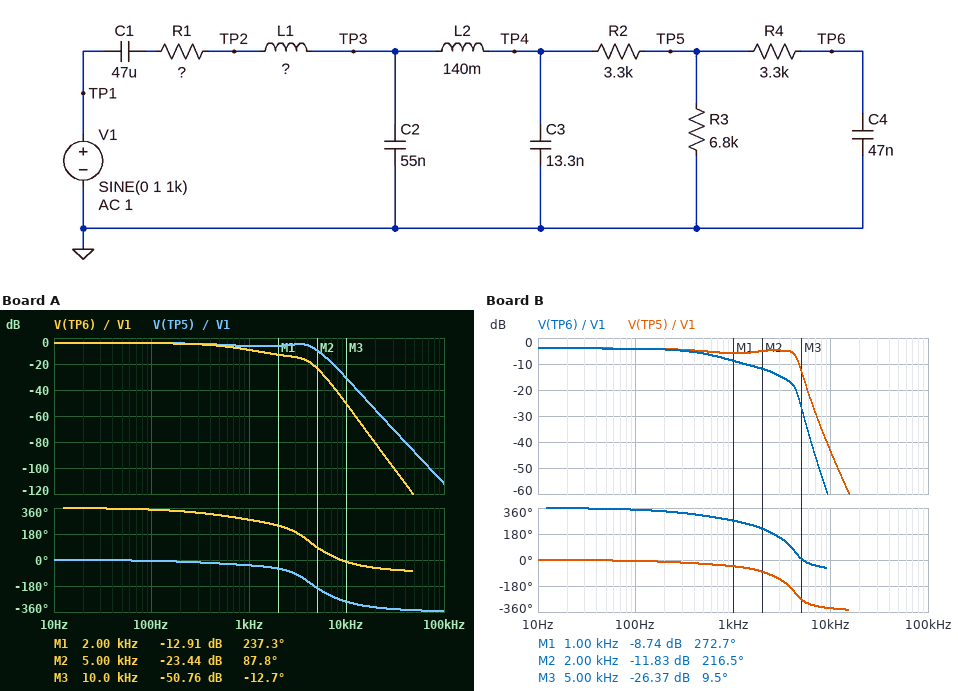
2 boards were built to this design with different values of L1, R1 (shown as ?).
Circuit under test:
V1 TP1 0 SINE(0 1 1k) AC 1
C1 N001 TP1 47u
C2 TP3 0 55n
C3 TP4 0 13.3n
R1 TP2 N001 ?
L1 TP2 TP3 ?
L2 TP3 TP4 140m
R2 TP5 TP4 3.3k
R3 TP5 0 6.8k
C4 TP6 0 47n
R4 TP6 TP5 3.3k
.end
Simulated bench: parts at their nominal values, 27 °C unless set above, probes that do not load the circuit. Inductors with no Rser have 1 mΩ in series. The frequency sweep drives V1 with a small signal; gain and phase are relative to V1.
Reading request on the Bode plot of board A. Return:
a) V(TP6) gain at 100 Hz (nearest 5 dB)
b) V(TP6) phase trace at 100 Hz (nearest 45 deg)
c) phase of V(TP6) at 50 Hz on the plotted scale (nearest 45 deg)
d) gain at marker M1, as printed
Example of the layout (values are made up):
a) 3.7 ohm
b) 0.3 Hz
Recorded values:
a) -5 dB
b) 360 deg
c) 360 deg
d) -12.91 dB
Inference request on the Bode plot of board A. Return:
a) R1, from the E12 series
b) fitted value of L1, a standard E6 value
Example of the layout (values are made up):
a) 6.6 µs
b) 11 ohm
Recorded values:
a) 560 Ω
b) 10 mH
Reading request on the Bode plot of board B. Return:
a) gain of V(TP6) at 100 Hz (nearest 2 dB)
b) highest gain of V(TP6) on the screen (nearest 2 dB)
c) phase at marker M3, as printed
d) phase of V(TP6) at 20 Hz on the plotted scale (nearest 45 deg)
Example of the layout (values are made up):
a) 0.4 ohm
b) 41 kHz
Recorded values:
a) -4 dB
b) -4 dB
c) 9.5 deg
d) 360 deg
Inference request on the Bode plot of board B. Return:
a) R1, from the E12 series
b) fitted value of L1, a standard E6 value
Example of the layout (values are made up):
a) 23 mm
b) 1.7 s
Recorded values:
a) 680 Ω
b) 47 mH
